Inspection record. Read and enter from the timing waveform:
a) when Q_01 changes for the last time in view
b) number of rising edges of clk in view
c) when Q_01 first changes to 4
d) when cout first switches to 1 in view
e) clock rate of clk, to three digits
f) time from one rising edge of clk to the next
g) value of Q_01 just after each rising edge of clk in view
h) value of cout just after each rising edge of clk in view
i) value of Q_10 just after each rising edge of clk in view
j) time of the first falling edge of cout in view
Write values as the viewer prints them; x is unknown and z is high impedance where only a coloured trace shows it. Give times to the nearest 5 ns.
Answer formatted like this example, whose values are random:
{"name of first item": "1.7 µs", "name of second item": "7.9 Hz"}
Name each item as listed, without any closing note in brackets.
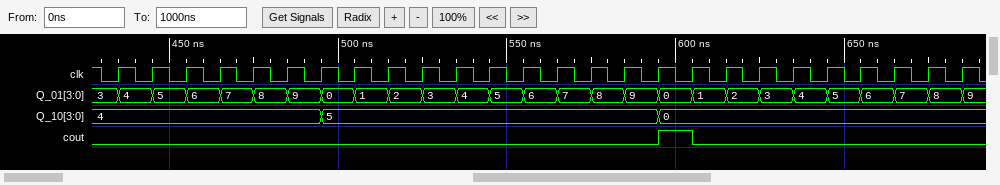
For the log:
{"when Q_01 changes for the last time in view": "685 ns", "number of rising edges of clk in view": "26", "when Q_01 first changes to 4": "435 ns", "when cout first switches to 1 in view": "595 ns", "clock rate of clk, to three digits": "100 MHz", "time from one rising edge of clk to the next": "10 ns", "value of Q_01 just after each rising edge of clk in view": "4, 5, 6, 7, 8, 9, 0, 1, 2, 3, 4, 5, 6, 7, 8, 9, 0, 1, 2, 3, 4, 5, 6, 7, 8, 9", "value of cout just after each rising edge of clk in view": "0 0 0 0 0 0 0 0 0 0 0 0 0 0 0 0 1 0 0 0 0 0 0 0 0 0", "value of Q_10 just after each rising edge of clk in view": "4, 4, 4, 4, 4, 4, 5, 5, 5, 5, 5, 5, 5, 5, 5, 5, 0, 0, 0, 0, 0, 0, 0, 0, 0, 0", "time of the first falling edge of cout in view": "605 ns"}
